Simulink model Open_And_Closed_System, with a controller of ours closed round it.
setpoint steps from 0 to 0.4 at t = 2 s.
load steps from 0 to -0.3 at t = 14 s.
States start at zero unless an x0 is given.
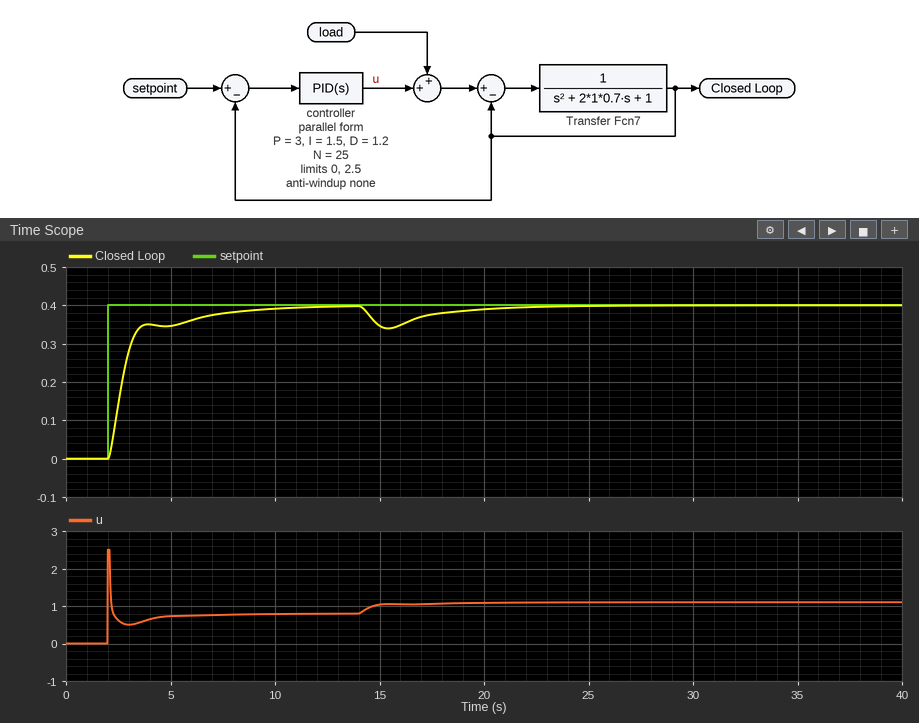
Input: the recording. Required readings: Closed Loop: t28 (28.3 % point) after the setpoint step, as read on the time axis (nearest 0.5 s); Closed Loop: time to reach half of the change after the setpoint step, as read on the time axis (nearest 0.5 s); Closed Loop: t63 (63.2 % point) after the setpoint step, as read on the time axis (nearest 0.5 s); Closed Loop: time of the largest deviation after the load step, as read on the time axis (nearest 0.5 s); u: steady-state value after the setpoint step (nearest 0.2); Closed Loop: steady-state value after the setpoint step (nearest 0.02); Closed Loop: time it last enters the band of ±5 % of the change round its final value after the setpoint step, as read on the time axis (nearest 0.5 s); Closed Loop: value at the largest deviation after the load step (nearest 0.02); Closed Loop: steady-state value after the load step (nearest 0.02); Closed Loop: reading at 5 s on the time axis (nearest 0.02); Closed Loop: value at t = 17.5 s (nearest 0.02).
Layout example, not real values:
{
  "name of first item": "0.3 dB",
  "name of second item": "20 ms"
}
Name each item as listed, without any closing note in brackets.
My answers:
{
  "Closed Loop: t28 (28.3 % point) after the setpoint step, as read on the time axis": "2.5 s",
  "Closed Loop: time to reach half of the change after the setpoint step, as read on the time axis": "2.5 s",
  "Closed Loop: t63 (63.2 % point) after the setpoint step, as read on the time axis": "3.0 s",
  "Closed Loop: time of the largest deviation after the load step, as read on the time axis": "15.5 s",
  "u: steady-state value after the setpoint step": "0.8",
  "Closed Loop: steady-state value after the setpoint step": "0.40",
  "Closed Loop: time it last enters the band of ±5 % of the change round its final value after the setpoint step, as read on the time axis": "7.5 s",
  "Closed Loop: value at the largest deviation after the load step": "0.34",
  "Closed Loop: steady-state value after the load step": "0.40",
  "Closed Loop: reading at 5 s on the time axis": "0.34",
  "Closed Loop: value at t = 17.5 s": "0.38"
}
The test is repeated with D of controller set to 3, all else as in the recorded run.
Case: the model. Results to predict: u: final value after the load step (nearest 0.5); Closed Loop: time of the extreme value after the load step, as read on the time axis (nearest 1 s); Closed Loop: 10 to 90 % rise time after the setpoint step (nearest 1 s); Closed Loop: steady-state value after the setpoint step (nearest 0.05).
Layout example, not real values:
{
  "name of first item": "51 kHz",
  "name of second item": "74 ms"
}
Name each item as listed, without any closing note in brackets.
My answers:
{
  "u: final value after the load step": "1.0",
  "Closed Loop: time of the extreme value after the load step, as read on the time axis": "16 s",
  "Closed Loop: 10 to 90 % rise time after the setpoint step": "3 s",
  "Closed Loop: steady-state value after the setpoint step": "0.40"
}
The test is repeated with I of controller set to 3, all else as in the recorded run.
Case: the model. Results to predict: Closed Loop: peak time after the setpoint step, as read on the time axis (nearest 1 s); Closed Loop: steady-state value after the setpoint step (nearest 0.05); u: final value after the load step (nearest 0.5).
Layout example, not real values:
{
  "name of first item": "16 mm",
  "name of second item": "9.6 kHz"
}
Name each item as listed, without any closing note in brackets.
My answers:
{
  "Closed Loop: peak time after the setpoint step, as read on the time axis": "4 s",
  "Closed Loop: steady-state value after the setpoint step": "0.40",
  "u: final value after the load step": "1.0"
}
